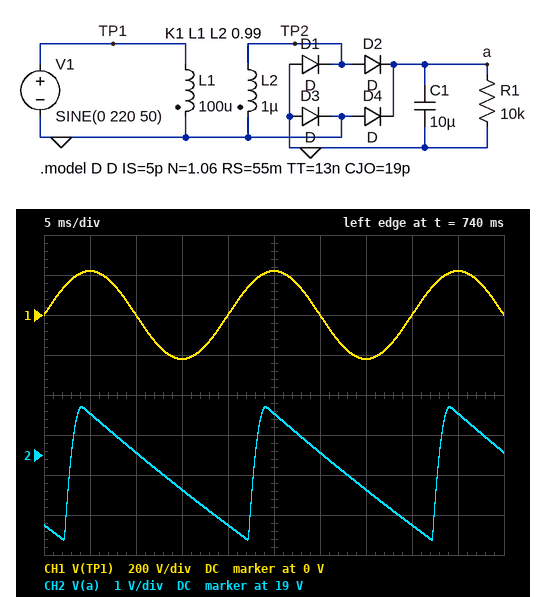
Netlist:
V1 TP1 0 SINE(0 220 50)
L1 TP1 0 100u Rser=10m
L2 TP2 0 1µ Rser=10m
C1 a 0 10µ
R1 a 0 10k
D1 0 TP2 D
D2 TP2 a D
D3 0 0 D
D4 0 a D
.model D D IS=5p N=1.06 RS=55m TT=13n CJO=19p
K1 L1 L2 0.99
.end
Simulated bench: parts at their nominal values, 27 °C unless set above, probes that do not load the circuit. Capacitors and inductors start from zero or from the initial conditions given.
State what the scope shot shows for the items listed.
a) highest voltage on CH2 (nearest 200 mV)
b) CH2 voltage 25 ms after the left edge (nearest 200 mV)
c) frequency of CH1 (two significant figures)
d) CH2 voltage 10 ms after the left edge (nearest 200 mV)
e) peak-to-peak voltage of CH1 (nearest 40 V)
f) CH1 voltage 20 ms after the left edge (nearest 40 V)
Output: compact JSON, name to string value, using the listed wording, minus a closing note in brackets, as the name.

{"highest voltage on CH2": "20.2 V", "CH2 voltage 25 ms after the left edge": "20.0 V", "frequency of CH1": "50 Hz", "CH2 voltage 10 ms after the left edge": "19.0 V", "peak-to-peak voltage of CH1": "440 V", "CH1 voltage 20 ms after the left edge": "0 V"}
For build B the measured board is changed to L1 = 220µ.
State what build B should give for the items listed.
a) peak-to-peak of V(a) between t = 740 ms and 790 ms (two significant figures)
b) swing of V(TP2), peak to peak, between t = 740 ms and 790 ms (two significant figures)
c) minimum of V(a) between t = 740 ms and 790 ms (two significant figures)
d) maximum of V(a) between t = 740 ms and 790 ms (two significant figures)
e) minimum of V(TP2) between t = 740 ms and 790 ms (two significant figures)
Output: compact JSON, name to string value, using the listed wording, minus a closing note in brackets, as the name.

{"peak-to-peak of V(a) between t = 740 ms and 790 ms": "2.3 V", "swing of V(TP2), peak to peak, between t = 740 ms and 790 ms": "27 V", "minimum of V(a) between t = 740 ms and 790 ms": "12 V", "maximum of V(a) between t = 740 ms and 790 ms": "14 V", "minimum of V(TP2) between t = 740 ms and 790 ms": "-12 V"}
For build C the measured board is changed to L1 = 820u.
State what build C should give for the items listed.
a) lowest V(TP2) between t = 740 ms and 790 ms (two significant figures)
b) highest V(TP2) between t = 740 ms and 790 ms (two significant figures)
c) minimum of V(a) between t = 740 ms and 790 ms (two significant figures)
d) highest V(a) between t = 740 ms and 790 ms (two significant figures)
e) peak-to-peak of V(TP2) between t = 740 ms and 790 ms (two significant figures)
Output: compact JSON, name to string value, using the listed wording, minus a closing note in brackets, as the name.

{"lowest V(TP2) between t = 740 ms and 790 ms": "-6.6 V", "highest V(TP2) between t = 740 ms and 790 ms": "7.6 V", "minimum of V(a) between t = 740 ms and 790 ms": "5.9 V", "highest V(a) between t = 740 ms and 790 ms": "7.1 V", "peak-to-peak of V(TP2) between t = 740 ms and 790 ms": "14 V"}
